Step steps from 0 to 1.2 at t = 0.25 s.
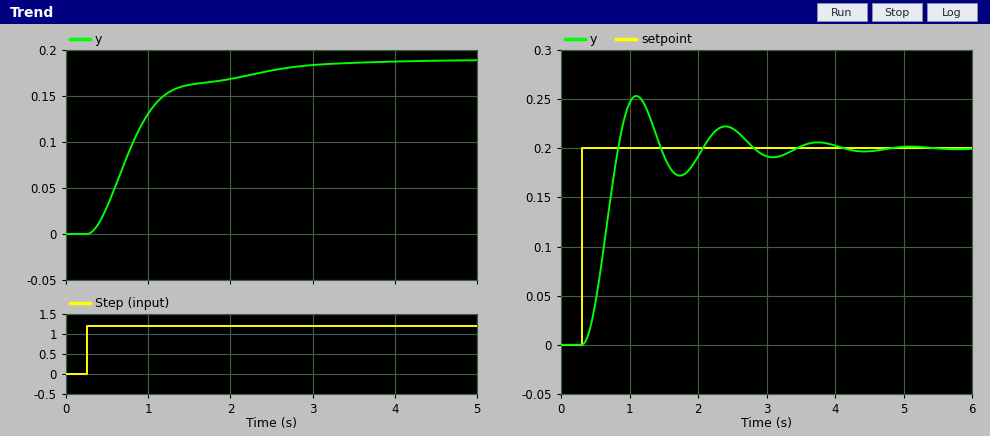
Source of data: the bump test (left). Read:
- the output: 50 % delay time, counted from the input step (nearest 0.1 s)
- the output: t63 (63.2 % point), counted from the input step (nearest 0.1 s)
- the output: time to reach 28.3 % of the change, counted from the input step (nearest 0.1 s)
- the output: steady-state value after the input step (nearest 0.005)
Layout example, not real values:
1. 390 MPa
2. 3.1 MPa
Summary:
1. 0.5 s
2. 0.7 s
3. 0.4 s
4. 0.190
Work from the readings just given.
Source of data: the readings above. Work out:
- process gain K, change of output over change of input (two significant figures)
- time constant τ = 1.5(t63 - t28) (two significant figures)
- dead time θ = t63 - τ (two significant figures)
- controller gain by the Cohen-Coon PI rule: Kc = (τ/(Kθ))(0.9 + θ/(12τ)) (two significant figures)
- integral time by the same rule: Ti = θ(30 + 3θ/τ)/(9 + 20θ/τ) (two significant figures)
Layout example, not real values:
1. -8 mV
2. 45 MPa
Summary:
1. 0.16
2. 0.45 s
3. 0.25 s
4. 11
5. 0.39 s
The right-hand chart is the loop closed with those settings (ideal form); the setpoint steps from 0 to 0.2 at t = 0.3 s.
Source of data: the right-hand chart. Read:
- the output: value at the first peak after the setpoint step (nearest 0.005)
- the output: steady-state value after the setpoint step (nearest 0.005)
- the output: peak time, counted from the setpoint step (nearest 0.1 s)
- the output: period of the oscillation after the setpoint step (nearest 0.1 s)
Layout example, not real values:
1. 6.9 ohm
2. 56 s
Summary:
1. 0.255
2. 0.200
3. 0.8 s
4. 1.3 s
